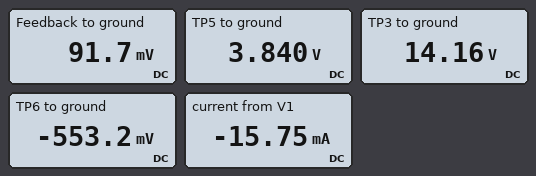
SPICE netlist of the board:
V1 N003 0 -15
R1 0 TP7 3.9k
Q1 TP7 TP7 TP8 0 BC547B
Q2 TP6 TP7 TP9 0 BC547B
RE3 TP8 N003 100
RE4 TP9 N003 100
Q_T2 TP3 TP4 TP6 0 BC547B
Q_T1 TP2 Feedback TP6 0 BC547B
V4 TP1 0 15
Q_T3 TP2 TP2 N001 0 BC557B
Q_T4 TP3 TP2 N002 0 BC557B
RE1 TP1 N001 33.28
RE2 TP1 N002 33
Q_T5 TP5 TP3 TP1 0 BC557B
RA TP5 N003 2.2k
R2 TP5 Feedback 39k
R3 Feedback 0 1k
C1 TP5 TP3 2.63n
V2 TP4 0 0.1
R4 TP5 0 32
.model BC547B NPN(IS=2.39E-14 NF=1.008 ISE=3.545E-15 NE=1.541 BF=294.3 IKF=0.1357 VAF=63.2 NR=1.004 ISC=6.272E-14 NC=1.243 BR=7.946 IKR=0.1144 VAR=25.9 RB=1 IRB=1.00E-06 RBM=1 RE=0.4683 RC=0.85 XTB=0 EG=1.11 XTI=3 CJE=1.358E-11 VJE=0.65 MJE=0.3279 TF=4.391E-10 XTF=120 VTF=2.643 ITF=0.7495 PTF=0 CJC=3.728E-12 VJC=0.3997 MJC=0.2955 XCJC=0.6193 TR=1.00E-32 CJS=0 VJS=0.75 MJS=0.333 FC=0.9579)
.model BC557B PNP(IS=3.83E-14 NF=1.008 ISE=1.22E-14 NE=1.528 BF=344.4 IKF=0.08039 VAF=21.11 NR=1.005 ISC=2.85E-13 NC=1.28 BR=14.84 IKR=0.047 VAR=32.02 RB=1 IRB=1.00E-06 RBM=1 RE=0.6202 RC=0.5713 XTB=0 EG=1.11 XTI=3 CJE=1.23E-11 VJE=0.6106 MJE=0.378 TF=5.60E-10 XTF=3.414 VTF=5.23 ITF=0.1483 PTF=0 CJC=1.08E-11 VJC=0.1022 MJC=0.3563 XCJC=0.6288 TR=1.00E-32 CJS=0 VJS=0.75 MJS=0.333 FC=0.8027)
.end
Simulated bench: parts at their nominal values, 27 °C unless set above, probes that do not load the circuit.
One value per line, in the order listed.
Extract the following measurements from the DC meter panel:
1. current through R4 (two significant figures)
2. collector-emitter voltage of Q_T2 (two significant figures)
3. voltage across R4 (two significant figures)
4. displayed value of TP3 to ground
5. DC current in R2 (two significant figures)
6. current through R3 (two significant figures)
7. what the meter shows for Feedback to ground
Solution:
120 mA
15 V
3.8 V
14.16 V
96 µA
92 µA
91.7 mV
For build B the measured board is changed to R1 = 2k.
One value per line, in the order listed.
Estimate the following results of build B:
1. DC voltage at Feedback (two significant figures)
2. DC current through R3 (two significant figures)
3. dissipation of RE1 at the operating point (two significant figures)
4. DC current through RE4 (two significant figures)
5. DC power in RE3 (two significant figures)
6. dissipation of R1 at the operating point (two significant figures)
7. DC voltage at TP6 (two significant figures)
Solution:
95 mV
95 µA
320 µW
6.8 mA
4.6 mW
93 mW
-570 mV
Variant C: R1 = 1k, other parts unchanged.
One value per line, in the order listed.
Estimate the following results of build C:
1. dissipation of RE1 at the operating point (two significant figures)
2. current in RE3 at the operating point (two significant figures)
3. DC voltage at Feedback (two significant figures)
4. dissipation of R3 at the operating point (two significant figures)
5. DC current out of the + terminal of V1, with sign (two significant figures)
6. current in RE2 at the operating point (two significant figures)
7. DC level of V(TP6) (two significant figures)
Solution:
1.2 mW
13 mA
97 mV
9.3 µW
-35 mA
6.1 mA
-590 mV
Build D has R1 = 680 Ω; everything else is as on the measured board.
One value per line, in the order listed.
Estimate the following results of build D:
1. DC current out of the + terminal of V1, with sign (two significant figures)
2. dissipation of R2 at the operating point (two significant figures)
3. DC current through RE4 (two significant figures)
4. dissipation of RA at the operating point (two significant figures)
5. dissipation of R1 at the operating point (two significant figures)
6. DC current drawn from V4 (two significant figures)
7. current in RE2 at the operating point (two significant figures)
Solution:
-46 mA
590 µW
18 mA
180 mW
230 mW
180 mA
8.7 mA
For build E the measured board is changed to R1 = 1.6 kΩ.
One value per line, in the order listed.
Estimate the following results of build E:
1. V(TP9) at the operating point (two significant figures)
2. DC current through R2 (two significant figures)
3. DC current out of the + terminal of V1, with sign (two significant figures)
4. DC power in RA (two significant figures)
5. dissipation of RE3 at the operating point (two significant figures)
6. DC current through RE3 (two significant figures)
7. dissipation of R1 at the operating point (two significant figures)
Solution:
-14 V
110 µA
-26 mA
170 mW
7.0 mW
8.4 mA
110 mW
